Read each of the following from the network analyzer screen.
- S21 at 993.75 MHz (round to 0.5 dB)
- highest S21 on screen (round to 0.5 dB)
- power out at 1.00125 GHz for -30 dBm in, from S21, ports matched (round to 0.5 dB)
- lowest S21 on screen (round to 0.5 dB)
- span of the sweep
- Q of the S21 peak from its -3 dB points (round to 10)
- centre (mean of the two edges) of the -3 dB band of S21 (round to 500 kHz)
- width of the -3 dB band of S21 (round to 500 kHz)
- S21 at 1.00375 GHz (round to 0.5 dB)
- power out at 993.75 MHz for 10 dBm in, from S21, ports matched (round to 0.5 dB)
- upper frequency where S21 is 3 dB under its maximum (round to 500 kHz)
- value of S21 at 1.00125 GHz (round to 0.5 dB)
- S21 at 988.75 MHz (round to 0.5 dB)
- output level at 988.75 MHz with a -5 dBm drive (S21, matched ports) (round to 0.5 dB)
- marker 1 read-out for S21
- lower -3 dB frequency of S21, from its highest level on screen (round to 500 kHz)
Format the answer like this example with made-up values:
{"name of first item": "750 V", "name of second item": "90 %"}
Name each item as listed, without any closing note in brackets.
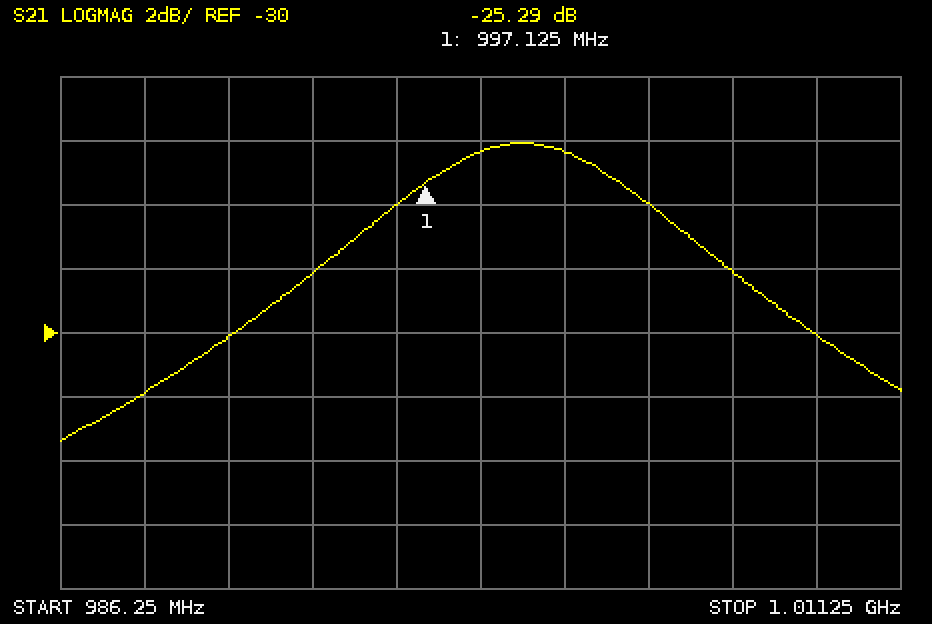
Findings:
{"S21 at 993.75 MHz": "-28.0 dB", "highest S21 on screen": "-24.0 dB", "power out at 1.00125 GHz for -30 dBm in, from S21, ports matched": "-54.5 dBm", "lowest S21 on screen": "-33.5 dB", "span of the sweep": "25 MHz", "Q of the S21 peak from its -3 dB points": "100", "centre (mean of the two edges) of the -3 dB band of S21": "1.0000 GHz", "width of the -3 dB band of S21": "10.0 MHz", "S21 at 1.00375 GHz": "-26.0 dB", "power out at 993.75 MHz for 10 dBm in, from S21, ports matched": "-18.0 dBm", "upper frequency where S21 is 3 dB under its maximum": "1.0050 GHz", "value of S21 at 1.00125 GHz": "-24.5 dB", "S21 at 988.75 MHz": "-32.0 dB", "output level at 988.75 MHz with a -5 dBm drive (S21, matched ports)": "-37.0 dBm", "marker 1 read-out for S21": "-25.29 dB", "lower -3 dB frequency of S21, from its highest level on screen": "995.0 MHz"}
